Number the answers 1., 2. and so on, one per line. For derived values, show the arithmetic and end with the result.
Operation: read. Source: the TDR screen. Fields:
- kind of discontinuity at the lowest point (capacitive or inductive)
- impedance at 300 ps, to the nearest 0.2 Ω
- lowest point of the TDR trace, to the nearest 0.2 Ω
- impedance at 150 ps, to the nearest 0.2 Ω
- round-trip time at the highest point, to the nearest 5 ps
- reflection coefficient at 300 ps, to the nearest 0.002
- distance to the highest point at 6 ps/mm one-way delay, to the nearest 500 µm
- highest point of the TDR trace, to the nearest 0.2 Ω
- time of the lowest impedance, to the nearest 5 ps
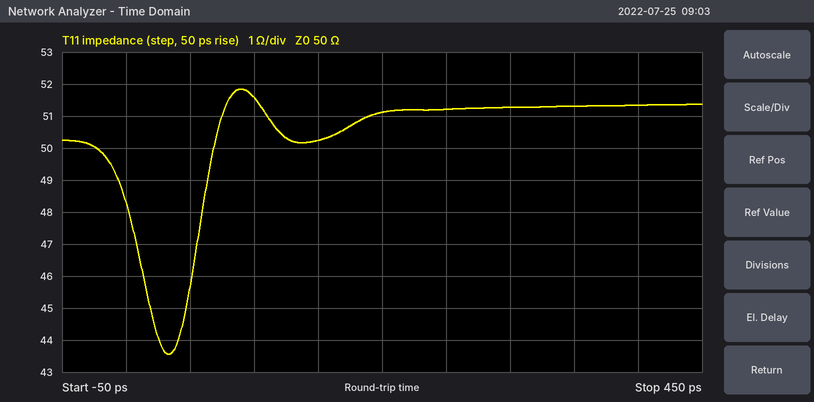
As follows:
1. capacitive
2. 51.2 Ω
3. 43.6 Ω
4. 50.2 Ω
5. 90 ps
6. (51.2 − 50)/(51.2 + 50) ≈ +0.012
7. 90 ps / 2 / 6 ps/mm ≈ 7.5 mm
8. 51.8 Ω
9. 35 ps
